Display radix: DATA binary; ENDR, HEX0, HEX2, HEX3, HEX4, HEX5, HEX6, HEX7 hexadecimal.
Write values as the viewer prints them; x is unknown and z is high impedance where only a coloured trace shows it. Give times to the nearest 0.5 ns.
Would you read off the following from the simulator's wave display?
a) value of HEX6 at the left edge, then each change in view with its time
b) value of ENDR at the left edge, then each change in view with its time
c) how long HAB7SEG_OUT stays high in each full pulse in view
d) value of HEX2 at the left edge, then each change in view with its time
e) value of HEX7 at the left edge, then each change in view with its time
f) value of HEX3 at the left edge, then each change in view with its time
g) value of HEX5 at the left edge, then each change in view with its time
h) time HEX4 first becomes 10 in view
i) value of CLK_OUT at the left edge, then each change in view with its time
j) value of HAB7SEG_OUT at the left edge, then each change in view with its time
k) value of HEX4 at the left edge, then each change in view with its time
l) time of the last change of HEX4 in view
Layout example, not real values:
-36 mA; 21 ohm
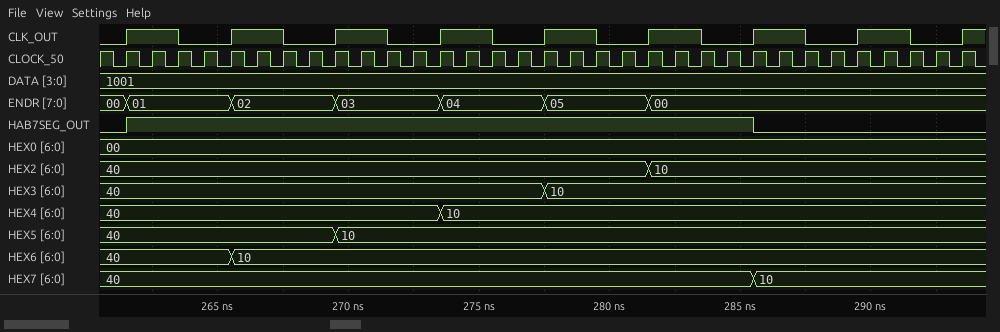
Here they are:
40, 10 at 265.5 ns; 00, 01 at 261.5 ns, 02 at 265.5 ns, 03 at 269.5 ns, 04 at 273.5 ns, 05 at 277.5 ns, 00 at 281.5 ns; 24 ns; 40, 10 at 281.5 ns; 40, 10 at 285.5 ns; 40, 10 at 277.5 ns; 40, 10 at 269.5 ns; 273.5 ns; 0, 1 at 261.5 ns, 0 at 263.5 ns, 1 at 265.5 ns, 0 at 267.5 ns, 1 at 269.5 ns, 0 at 271.5 ns, 1 at 273.5 ns, 0 at 275.5 ns, 1 at 277.5 ns, 0 at 279.5 ns, 1 at 281.5 ns, 0 at 283.5 ns, 1 at 285.5 ns, 0 at 287.5 ns, 1 at 289.5 ns, 0 at 291.5 ns, 1 at 293.5 ns; 0, 1 at 261.5 ns, 0 at 285.5 ns; 40, 10 at 273.5 ns; 273.5 ns
